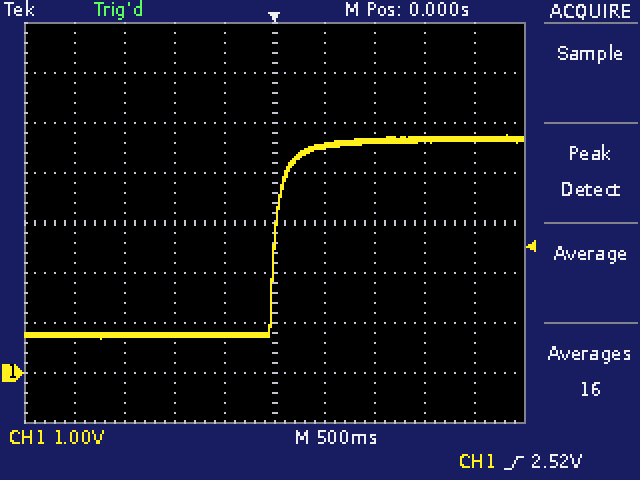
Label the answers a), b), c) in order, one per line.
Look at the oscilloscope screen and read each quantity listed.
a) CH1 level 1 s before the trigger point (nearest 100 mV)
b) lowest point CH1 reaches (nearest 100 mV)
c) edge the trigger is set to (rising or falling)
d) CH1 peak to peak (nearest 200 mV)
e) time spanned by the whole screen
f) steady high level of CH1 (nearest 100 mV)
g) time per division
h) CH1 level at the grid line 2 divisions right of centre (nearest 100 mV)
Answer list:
a) 800 mV
b) 700 mV
c) rising
d) 4.0 V
e) 5 s
f) 4.7 V
g) 500 ms
h) 4.6 V
